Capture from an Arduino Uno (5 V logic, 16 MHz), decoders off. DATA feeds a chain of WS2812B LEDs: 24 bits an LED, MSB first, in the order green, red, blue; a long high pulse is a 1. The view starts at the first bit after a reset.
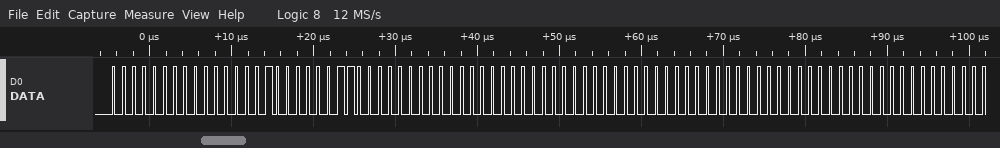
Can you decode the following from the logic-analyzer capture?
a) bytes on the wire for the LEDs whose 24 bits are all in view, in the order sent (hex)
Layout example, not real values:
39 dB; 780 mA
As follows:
00 01 03 00 00 00 00 00 00
